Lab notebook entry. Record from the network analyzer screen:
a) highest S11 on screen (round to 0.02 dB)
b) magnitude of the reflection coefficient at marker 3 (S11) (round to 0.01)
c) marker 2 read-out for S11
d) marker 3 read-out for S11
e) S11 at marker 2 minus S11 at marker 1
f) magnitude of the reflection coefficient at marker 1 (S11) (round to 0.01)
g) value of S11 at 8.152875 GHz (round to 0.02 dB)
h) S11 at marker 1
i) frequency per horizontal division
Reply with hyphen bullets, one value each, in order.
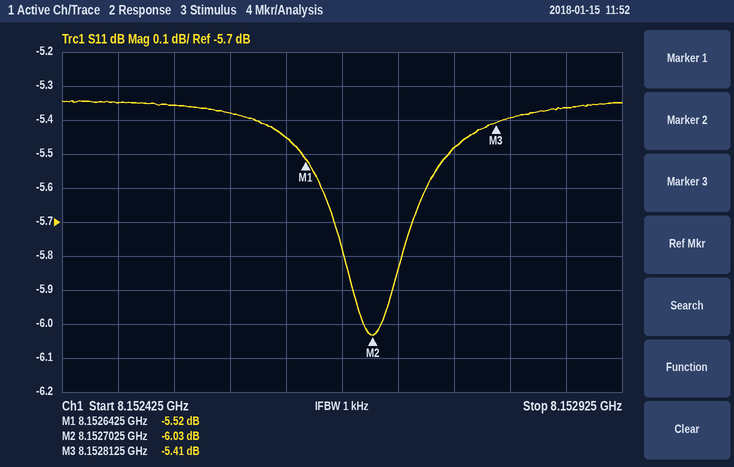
- -5.34 dB
- 0.54
- -6.03 dB
- -5.41 dB
- -0.51 dB
- 0.53
- -5.36 dB
- -5.52 dB
- 50 kHz
